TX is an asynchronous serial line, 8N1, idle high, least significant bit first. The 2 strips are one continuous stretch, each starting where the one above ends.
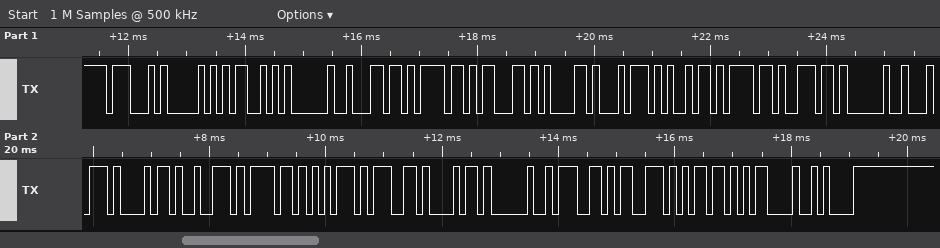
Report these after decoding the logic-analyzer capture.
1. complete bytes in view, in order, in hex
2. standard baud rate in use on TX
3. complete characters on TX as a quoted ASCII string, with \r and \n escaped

47 50 53 20 6C 6F 63 61 74 69 6F 6E 20 74 68 72 6F 75 67 68 20 67 73 6D 0D 0A
9600 baud
"GPS location through gsm\r\n"
